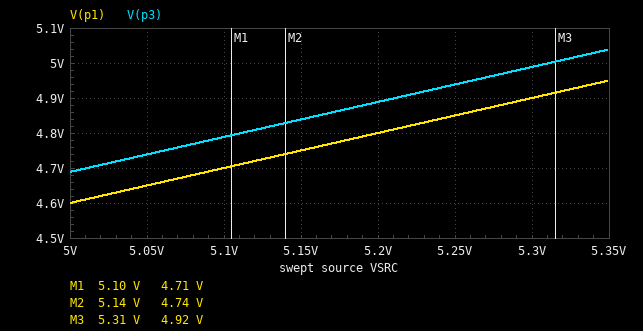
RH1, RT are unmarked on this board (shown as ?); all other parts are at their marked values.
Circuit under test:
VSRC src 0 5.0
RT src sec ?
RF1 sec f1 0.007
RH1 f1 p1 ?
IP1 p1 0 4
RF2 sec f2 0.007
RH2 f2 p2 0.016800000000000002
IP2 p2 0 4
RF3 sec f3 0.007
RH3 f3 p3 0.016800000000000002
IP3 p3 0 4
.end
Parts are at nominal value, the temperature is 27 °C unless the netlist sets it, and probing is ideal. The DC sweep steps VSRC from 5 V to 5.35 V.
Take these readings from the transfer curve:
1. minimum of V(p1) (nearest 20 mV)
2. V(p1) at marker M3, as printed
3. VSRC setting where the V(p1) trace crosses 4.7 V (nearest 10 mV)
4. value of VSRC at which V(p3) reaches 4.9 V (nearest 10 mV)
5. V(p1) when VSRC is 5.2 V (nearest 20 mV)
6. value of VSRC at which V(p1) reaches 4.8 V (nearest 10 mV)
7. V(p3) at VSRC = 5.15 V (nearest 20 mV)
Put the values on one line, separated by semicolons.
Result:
4.60 V; 4.92 V; 5.10 V; 5.21 V; 4.80 V; 5.20 V; 4.84 V
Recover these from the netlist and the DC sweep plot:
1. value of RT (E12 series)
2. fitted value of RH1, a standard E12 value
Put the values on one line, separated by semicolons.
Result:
0.018 Ω; 0.039 Ω
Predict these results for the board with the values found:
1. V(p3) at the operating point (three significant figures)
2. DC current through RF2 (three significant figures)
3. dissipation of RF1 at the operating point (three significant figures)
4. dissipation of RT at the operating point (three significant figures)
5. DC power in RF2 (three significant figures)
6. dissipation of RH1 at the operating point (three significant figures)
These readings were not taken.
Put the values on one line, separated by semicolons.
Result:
4.69 V; 4.00 A; 112 mW; 2.59 W; 112 mW; 624 mW
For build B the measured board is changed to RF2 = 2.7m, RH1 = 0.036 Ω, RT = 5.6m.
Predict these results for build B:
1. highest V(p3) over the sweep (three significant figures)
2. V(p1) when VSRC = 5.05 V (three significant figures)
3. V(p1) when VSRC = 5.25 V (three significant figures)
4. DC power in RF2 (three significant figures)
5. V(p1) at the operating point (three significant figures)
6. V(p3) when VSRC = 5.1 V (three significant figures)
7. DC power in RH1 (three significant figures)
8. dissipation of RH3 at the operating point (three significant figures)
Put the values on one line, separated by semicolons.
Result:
5.19 V; 4.81 V; 5.01 V; 43.2 mW; 4.76 V; 4.94 V; 576 mW; 269 mW
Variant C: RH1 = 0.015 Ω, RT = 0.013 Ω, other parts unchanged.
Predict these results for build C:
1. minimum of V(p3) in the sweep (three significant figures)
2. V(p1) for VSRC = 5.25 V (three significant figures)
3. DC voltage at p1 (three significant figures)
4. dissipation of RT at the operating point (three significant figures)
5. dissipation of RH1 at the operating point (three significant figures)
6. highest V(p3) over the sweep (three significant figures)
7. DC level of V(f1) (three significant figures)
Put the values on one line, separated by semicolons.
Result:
4.75 V; 5.01 V; 4.76 V; 1.87 W; 240 mW; 5.10 V; 4.82 V
